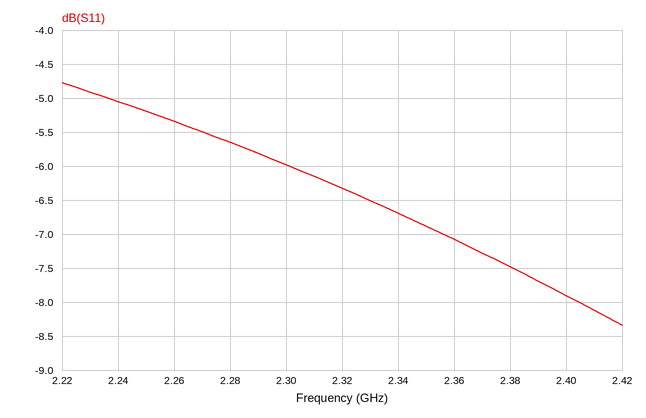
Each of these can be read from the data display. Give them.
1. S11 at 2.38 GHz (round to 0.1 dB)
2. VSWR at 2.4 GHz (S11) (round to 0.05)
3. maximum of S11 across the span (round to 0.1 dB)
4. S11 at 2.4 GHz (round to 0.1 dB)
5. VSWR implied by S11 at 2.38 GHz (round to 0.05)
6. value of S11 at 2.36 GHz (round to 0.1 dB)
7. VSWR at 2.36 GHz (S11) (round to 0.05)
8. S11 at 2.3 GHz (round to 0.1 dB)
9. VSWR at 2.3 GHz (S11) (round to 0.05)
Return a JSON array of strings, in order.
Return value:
["-7.5 dB", "2.35", "-4.8 dB", "-7.9 dB", "2.45", "-7.1 dB", "2.60", "-6.0 dB", "3.00"]
